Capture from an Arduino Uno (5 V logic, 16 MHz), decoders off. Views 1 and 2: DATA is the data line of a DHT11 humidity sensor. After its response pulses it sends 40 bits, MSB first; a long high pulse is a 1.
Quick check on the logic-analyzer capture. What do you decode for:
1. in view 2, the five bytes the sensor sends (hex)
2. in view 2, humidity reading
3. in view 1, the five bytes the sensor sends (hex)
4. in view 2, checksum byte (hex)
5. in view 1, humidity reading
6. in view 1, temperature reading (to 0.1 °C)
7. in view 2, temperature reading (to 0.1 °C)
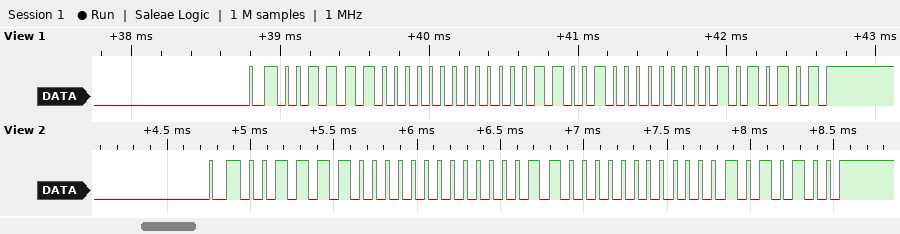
3C 00 18 00 54
60 %
3C 00 19 00 55
0x54
60 %
25.0 °C
24.0 °C
